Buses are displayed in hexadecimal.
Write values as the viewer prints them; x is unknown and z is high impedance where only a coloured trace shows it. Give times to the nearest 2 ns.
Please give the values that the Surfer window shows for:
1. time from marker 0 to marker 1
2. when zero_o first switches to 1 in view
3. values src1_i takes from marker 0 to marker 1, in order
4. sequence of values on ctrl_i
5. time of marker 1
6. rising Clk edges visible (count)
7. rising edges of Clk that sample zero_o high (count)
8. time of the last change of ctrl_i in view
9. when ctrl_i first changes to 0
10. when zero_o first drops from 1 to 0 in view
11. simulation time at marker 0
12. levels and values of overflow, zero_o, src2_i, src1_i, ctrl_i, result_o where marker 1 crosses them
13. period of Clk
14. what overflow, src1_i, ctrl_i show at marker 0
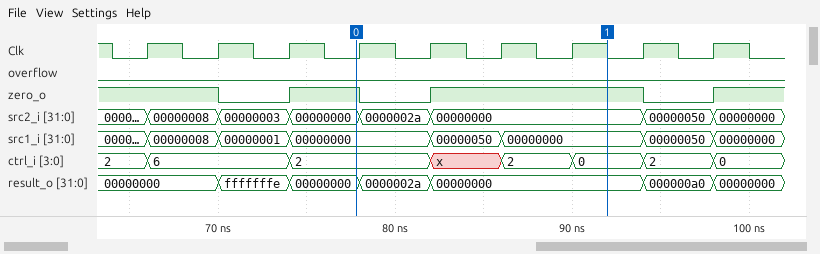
14 ns
74 ns
00000000, 00000050, 00000000
2, 6, 2, x, 2, 0, 2, 0
92 ns
9
6
98 ns
90 ns
70 ns
78 ns
overflow=0, zero_o=1, src2_i=00000000, src1_i=00000000, ctrl_i=0, result_o=00000000
4 ns
overflow=0, src1_i=00000000, ctrl_i=2
